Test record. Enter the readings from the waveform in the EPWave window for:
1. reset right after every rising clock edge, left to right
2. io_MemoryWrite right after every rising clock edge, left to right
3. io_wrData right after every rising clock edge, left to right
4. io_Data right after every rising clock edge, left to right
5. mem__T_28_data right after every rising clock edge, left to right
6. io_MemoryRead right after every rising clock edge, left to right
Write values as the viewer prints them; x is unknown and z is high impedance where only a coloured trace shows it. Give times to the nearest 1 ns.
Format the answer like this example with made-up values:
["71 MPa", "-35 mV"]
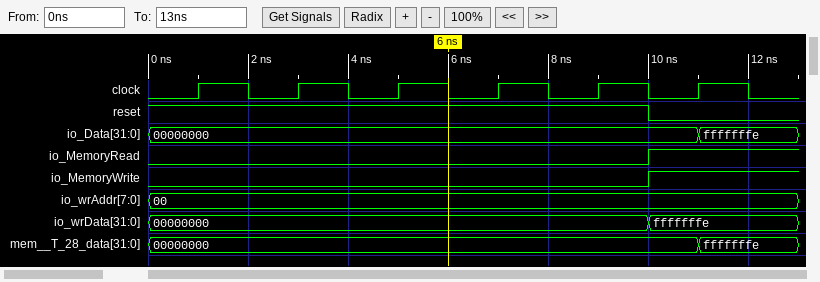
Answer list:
["1 1 1 1 1 0", "0 0 0 0 0 1", "00000000, 00000000, 00000000, 00000000, 00000000, fffffffe", "00000000, 00000000, 00000000, 00000000, 00000000, fffffffe", "00000000, 00000000, 00000000, 00000000, 00000000, fffffffe", "0 0 0 0 0 1"]
